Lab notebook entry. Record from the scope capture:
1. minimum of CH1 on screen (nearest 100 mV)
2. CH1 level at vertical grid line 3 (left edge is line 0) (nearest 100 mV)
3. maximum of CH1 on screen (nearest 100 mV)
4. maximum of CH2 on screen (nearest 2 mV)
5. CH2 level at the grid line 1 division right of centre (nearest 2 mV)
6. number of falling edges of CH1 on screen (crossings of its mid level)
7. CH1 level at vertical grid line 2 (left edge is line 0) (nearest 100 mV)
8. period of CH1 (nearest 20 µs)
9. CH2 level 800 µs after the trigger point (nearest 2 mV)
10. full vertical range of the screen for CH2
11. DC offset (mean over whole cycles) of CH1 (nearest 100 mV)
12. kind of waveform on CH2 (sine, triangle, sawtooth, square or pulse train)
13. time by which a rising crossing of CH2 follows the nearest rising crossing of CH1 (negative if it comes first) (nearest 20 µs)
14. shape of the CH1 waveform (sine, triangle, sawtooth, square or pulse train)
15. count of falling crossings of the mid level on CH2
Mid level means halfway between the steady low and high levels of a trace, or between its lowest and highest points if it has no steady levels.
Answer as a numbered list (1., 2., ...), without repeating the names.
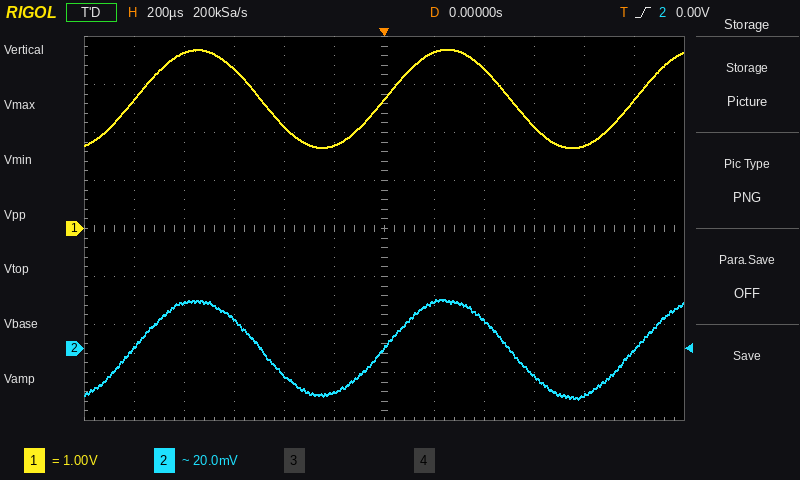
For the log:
1. 1.7 V
2. 3.3 V
3. 3.7 V
4. 20 mV
5. 20 mV
6. 2
7. 3.7 V
8. 1.00 ms
9. -20 mV
10. 160 mV
11. 2.7 V
12. sine
13. 0 µs
14. sine
15. 2
